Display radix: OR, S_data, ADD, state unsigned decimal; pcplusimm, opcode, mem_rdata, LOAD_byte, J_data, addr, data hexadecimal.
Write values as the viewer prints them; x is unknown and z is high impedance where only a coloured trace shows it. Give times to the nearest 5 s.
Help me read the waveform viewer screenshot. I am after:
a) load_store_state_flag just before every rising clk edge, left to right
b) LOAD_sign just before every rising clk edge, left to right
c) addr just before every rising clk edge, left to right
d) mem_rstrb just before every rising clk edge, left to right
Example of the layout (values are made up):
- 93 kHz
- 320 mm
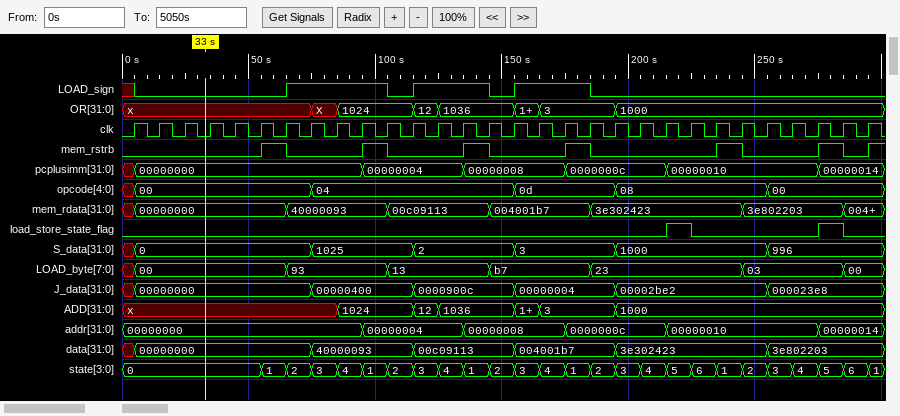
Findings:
- 0 0 0 0 0 0 0 0 0 0 0 0 0 0 0 0 0 0 0 0 0 0 1 0 0 0 0 0 1 0
- x 0 0 0 0 0 0 1 1 1 1 0 1 1 1 0 1 1 1 0 0 0 0 0 0 0 0 0 0 0
- 00000000, 00000000, 00000000, 00000000, 00000000, 00000000, 00000000, 00000000, 00000000, 00000000, 00000004, 00000004, 00000004, 00000004, 00000008, 00000008, 00000008, 00000008, 0000000c, 0000000c, 0000000c, 0000000c, 00000010, 00000010, 00000010, 00000010, 00000010, 00000010, 00000014, 00000014
- 0 0 0 0 0 0 1 0 0 0 1 0 0 0 1 0 0 0 1 0 0 0 0 0 1 0 0 0 1 0
